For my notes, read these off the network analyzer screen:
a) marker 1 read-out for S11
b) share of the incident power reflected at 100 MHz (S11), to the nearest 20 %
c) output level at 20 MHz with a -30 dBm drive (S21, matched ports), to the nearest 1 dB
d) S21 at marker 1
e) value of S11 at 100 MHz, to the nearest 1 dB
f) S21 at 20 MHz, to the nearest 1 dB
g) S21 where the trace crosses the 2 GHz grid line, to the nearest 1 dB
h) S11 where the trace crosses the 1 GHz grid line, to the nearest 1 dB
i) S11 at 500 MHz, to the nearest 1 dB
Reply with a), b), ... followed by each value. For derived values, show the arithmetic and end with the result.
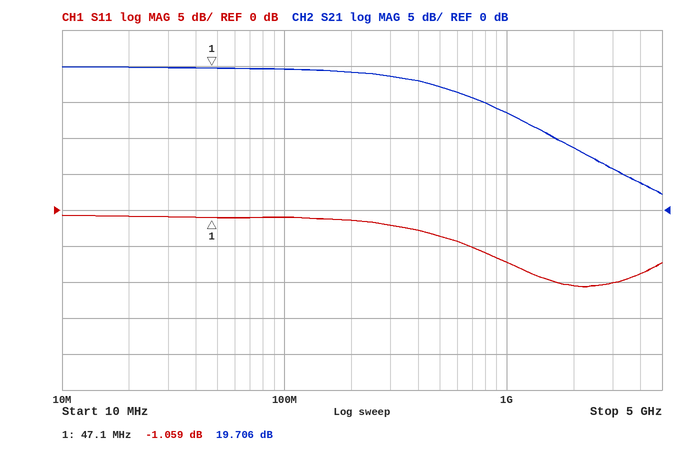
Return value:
a) -1.059 dB
b) 10^(-1/10) ≈ 79.4 %, so 80 % to the nearest 20 %
c) -30 dBm + (20 dB) = -10 dBm
d) 19.706 dB
e) -1 dB
f) 20 dB
g) 9 dB
h) -7 dB
i) -4 dB
